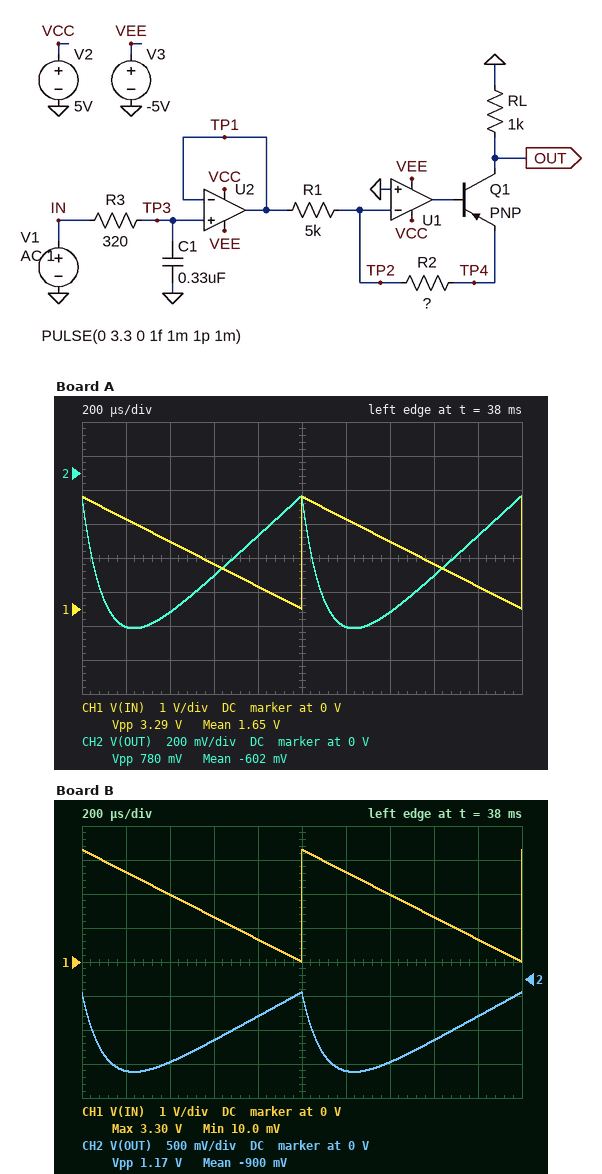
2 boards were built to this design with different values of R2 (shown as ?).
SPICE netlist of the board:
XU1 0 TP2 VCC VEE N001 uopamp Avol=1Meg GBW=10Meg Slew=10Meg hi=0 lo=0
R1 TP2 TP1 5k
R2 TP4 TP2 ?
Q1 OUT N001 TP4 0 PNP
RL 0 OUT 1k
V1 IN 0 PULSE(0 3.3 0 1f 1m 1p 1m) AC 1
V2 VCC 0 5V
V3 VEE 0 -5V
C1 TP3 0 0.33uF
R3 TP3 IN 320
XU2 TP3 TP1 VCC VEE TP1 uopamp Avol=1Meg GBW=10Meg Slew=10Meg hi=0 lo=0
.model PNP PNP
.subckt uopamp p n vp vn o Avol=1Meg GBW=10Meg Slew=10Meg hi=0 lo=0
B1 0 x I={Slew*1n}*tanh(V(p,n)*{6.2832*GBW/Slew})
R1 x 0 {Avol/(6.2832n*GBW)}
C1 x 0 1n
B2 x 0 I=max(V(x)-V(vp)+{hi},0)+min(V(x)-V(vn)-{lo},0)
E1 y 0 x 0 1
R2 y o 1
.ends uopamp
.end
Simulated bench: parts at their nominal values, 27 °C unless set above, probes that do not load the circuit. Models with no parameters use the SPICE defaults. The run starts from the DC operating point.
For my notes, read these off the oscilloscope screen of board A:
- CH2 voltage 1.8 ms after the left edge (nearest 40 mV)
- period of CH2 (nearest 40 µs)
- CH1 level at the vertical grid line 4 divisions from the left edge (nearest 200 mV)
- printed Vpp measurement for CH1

-360 mV
1.00 ms
600 mV
3.29 V
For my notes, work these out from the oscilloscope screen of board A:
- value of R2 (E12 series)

1.8 kΩ
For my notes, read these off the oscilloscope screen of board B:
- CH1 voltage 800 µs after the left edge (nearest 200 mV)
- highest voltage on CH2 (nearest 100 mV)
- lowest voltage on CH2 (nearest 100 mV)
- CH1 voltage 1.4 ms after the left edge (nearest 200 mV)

600 mV
-200 mV
-1.4 V
2.0 V
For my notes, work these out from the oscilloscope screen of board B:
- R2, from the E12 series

2.7 kΩ
